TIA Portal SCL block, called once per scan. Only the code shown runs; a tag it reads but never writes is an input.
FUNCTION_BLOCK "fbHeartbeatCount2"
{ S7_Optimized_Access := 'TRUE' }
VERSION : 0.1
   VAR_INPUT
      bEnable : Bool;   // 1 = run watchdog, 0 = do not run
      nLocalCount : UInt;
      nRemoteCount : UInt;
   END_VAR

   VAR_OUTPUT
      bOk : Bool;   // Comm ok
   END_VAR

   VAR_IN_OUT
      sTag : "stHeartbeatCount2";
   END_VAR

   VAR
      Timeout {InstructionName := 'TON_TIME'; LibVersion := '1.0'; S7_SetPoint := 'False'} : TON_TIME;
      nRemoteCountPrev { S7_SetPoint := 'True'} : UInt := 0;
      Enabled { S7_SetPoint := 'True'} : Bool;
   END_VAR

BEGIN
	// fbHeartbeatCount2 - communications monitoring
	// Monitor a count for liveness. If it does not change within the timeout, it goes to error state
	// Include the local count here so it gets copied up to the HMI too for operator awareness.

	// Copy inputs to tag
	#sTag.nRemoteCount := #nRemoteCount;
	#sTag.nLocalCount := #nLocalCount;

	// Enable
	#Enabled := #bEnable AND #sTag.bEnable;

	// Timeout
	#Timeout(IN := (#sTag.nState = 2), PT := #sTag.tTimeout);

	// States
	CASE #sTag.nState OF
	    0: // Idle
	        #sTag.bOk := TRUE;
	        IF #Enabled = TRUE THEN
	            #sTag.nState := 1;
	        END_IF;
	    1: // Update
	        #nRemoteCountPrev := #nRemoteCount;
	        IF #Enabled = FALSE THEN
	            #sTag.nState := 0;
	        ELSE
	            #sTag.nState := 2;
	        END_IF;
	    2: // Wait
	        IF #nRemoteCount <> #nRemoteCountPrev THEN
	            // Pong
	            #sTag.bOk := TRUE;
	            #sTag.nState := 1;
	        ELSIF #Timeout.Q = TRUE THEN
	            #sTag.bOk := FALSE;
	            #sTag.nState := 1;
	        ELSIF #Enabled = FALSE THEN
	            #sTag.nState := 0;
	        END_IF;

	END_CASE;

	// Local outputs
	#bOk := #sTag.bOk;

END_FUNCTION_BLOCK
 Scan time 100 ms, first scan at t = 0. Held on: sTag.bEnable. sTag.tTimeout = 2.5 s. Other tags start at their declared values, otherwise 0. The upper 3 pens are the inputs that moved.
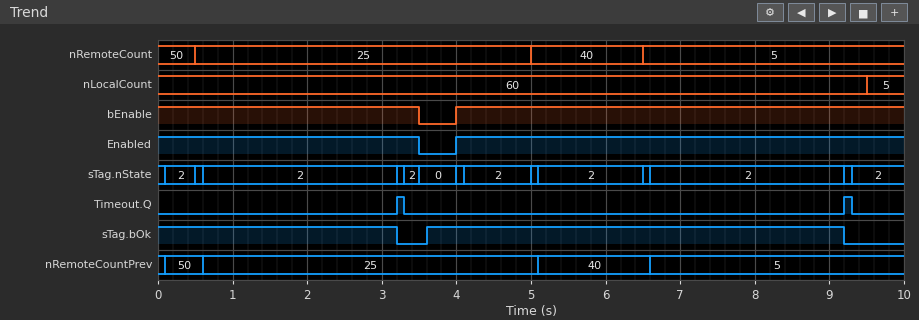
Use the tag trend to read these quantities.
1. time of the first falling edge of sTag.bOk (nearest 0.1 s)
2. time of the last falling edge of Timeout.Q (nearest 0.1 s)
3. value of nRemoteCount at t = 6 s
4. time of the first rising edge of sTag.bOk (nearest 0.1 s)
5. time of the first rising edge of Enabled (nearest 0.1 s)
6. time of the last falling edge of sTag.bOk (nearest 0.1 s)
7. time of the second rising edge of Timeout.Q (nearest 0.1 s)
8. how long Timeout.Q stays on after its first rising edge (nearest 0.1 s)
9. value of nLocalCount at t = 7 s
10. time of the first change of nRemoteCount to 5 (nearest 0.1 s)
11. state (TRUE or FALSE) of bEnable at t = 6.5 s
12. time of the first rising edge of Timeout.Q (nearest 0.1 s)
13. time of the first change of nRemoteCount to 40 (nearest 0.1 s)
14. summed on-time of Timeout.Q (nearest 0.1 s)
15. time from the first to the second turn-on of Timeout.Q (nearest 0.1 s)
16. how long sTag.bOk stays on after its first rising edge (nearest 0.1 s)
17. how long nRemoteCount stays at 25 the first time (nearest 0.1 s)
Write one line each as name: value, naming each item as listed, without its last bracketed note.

time of the first falling edge of sTag.bOk: 3.2 s
time of the last falling edge of Timeout.Q: 9.3 s
value of nRemoteCount at t = 6 s: 40
time of the first rising edge of sTag.bOk: 3.6 s
time of the first rising edge of Enabled: 4.0 s
time of the last falling edge of sTag.bOk: 9.2 s
time of the second rising edge of Timeout.Q: 9.2 s
how long Timeout.Q stays on after its first rising edge: 0.1 s
value of nLocalCount at t = 7 s: 60
time of the first change of nRemoteCount to 5: 6.5 s
state (TRUE or FALSE) of bEnable at t = 6.5 s: TRUE
time of the first rising edge of Timeout.Q: 3.2 s
time of the first change of nRemoteCount to 40: 5.0 s
summed on-time of Timeout.Q: 0.2 s
time from the first to the second turn-on of Timeout.Q: 6.0 s
how long sTag.bOk stays on after its first rising edge: 5.6 s
how long nRemoteCount stays at 25 the first time: 4.5 s
